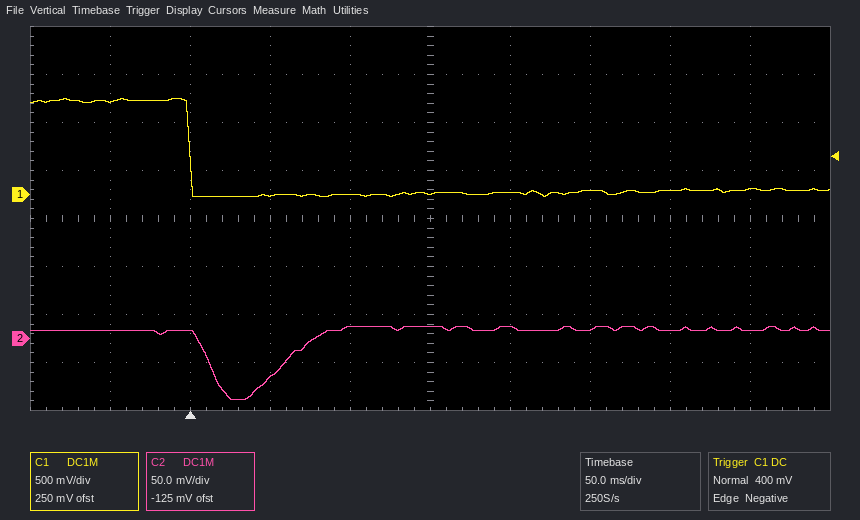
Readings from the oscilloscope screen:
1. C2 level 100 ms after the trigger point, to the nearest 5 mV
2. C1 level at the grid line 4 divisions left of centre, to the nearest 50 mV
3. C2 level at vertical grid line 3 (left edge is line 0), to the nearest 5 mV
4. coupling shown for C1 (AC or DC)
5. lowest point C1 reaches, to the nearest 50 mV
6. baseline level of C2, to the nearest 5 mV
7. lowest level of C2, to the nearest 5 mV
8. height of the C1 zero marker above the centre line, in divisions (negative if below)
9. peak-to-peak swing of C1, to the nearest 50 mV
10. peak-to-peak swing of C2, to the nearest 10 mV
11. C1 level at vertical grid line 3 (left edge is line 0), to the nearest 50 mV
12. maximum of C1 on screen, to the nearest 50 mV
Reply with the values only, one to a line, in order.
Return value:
10 mV
950 mV
-40 mV
DC
0 mV
10 mV
-65 mV
+0.5 div
1.00 V
80 mV
0 mV
1.00 V
